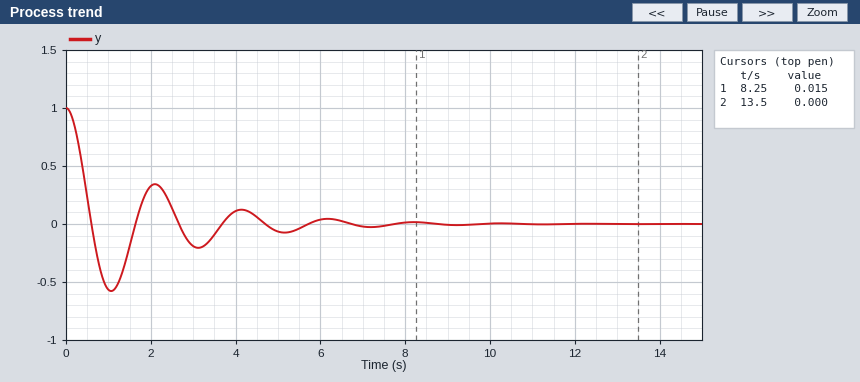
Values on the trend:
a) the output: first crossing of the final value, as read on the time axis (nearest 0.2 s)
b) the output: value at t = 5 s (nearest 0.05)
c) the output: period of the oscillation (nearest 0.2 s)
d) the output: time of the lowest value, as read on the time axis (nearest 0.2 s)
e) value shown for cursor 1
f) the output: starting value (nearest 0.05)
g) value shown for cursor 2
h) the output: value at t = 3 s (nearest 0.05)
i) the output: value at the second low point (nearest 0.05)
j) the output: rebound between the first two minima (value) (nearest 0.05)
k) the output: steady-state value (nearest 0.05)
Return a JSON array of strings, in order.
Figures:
["0.6 s", "-0.05", "2.0 s", "1.0 s", "0.015", "1.00", "0.000", "-0.20", "-0.20", "0.35", "0.00"]
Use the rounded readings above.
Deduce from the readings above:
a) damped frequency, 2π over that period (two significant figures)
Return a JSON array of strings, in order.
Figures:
["3.1 rad/s"]
